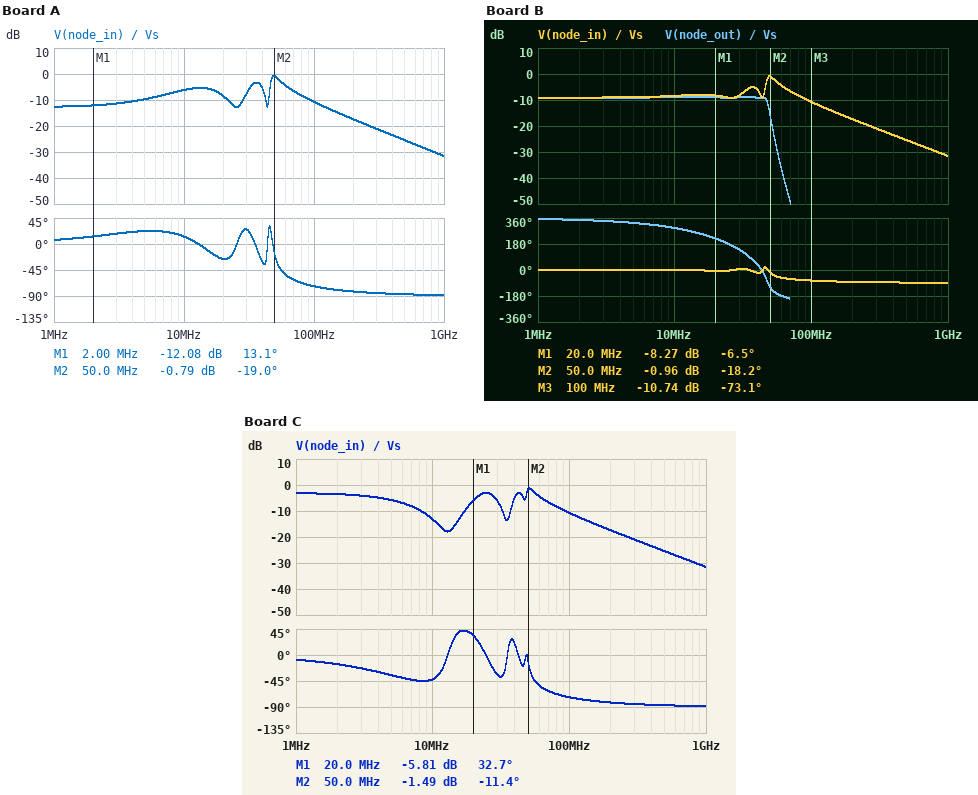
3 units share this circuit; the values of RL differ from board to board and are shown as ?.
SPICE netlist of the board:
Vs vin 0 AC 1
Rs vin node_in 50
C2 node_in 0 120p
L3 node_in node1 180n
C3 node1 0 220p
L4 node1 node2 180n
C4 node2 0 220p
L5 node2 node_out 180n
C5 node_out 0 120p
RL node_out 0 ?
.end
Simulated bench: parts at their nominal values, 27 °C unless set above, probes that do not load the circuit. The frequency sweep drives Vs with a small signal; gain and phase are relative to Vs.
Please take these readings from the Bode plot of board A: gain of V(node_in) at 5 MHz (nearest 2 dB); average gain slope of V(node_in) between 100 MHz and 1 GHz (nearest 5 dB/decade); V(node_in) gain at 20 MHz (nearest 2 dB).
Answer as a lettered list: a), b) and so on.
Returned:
a) -10 dB
b) -20 dB/decade
c) -8 dB
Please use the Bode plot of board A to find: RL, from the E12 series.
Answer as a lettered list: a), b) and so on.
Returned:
a) 15 Ω
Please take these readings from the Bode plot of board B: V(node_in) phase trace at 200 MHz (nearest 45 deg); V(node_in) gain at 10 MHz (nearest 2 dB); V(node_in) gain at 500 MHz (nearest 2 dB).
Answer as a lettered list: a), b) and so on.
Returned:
a) -90 deg
b) -8 dB
c) -26 dB
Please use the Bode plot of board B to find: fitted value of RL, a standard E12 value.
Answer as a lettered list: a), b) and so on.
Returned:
a) 27 Ω
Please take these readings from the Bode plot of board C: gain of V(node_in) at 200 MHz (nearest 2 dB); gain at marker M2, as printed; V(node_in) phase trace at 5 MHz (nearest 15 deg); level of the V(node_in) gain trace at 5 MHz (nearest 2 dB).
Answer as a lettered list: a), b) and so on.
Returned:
a) -18 dB
b) -1.49 dB
c) -30 deg
d) -6 dB
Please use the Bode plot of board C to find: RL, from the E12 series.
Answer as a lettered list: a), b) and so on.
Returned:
a) 120 Ω
